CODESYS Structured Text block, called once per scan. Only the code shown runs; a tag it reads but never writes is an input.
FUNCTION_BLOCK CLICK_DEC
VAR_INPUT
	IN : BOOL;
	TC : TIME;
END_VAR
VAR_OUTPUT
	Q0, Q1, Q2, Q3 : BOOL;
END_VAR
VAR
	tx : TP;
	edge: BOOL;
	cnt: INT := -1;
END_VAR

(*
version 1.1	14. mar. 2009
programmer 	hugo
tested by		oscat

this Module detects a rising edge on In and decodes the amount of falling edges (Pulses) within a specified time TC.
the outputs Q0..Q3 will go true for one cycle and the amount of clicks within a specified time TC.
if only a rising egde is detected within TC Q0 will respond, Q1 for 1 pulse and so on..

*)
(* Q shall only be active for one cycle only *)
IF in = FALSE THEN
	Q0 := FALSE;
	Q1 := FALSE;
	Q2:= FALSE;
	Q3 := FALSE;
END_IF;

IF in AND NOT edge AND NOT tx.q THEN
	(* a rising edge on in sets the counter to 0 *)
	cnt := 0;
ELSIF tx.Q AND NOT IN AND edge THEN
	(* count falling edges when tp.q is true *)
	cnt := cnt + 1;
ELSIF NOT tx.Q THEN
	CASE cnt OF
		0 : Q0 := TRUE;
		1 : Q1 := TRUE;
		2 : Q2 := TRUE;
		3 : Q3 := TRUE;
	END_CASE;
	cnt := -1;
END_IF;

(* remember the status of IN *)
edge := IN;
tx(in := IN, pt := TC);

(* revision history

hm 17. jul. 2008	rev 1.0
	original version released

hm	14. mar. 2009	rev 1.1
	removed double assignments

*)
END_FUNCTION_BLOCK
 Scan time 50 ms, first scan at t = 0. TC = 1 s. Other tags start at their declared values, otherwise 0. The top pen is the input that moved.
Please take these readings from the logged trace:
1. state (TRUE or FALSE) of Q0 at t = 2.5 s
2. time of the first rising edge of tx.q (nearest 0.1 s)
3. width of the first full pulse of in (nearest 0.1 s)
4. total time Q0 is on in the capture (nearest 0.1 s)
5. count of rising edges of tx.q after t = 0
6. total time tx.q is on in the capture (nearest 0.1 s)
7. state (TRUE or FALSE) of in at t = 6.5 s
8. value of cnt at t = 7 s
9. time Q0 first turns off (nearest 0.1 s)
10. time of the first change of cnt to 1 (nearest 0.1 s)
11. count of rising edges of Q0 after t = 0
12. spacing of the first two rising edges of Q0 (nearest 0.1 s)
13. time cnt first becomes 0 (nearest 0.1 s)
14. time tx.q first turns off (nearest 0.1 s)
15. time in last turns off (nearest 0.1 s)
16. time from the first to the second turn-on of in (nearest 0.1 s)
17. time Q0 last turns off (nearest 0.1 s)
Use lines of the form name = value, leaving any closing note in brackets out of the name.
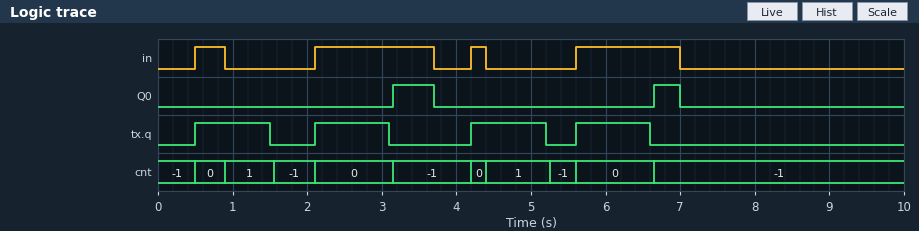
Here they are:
state (TRUE or FALSE) of Q0 at t = 2.5 s = FALSE
time of the first rising edge of tx.q = 0.5 s
width of the first full pulse of in = 0.4 s
total time Q0 is on in the capture = 0.9 s
count of rising edges of tx.q after t = 0 = 4
total time tx.q is on in the capture = 4.0 s
state (TRUE or FALSE) of in at t = 6.5 s = TRUE
value of cnt at t = 7 s = -1
time Q0 first turns off = 3.7 s
time of the first change of cnt to 1 = 0.9 s
count of rising edges of Q0 after t = 0 = 2
spacing of the first two rising edges of Q0 = 3.5 s
time cnt first becomes 0 = 0.5 s
time tx.q first turns off = 1.5 s
time in last turns off = 7.0 s
time from the first to the second turn-on of in = 1.6 s
time Q0 last turns off = 7.0 s
